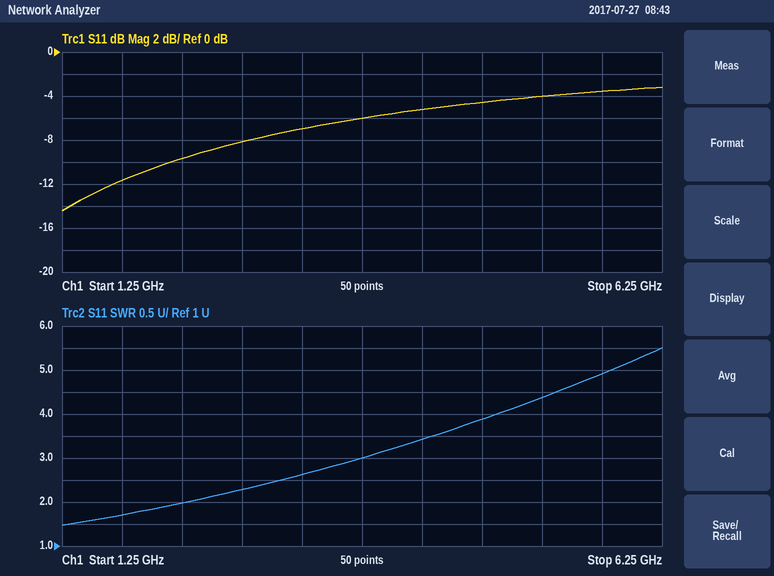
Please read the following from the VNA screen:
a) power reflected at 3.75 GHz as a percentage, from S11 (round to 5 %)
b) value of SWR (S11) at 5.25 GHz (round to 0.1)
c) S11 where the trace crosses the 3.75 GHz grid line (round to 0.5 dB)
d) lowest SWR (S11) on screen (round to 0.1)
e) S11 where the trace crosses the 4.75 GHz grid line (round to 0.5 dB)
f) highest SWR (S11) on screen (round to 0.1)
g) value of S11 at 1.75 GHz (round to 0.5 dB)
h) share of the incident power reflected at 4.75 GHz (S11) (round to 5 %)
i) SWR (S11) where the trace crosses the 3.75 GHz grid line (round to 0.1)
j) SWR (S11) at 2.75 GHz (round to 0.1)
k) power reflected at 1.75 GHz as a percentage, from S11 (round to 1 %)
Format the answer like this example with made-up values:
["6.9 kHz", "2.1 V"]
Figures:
["25 %", "4.4", "-6.0 dB", "1.5", "-4.5 dB", "5.5", "-11.5 dB", "35 %", "3.0", "2.3", "7 %"]
